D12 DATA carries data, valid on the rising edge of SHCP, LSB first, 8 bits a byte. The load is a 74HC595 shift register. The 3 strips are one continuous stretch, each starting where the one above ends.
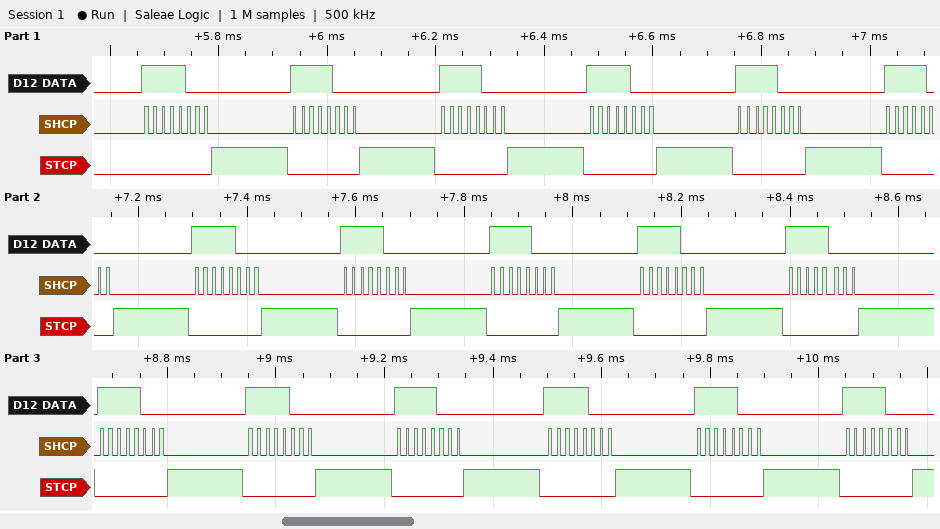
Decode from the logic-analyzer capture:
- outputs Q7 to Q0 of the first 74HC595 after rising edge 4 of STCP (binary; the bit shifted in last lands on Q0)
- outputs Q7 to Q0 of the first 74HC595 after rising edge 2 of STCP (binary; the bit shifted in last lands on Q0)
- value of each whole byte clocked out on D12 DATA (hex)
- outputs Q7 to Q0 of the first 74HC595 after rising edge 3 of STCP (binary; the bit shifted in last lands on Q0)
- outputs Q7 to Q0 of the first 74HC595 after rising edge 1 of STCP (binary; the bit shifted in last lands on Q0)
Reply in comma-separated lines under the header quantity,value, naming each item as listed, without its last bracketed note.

quantity,value
outputs Q7 to Q0 of the first 74HC595 after rising edge 4 of STCP,11111000
outputs Q7 to Q0 of the first 74HC595 after rising edge 2 of STCP,11111000
value of each whole byte clocked out on D12 DATA,1F 1F 1F 1F 1F 1F 1F 1F 1F 1F 1F 1F 1F 1F 1F 1F 1F
outputs Q7 to Q0 of the first 74HC595 after rising edge 3 of STCP,11111000
outputs Q7 to Q0 of the first 74HC595 after rising edge 1 of STCP,11111000
